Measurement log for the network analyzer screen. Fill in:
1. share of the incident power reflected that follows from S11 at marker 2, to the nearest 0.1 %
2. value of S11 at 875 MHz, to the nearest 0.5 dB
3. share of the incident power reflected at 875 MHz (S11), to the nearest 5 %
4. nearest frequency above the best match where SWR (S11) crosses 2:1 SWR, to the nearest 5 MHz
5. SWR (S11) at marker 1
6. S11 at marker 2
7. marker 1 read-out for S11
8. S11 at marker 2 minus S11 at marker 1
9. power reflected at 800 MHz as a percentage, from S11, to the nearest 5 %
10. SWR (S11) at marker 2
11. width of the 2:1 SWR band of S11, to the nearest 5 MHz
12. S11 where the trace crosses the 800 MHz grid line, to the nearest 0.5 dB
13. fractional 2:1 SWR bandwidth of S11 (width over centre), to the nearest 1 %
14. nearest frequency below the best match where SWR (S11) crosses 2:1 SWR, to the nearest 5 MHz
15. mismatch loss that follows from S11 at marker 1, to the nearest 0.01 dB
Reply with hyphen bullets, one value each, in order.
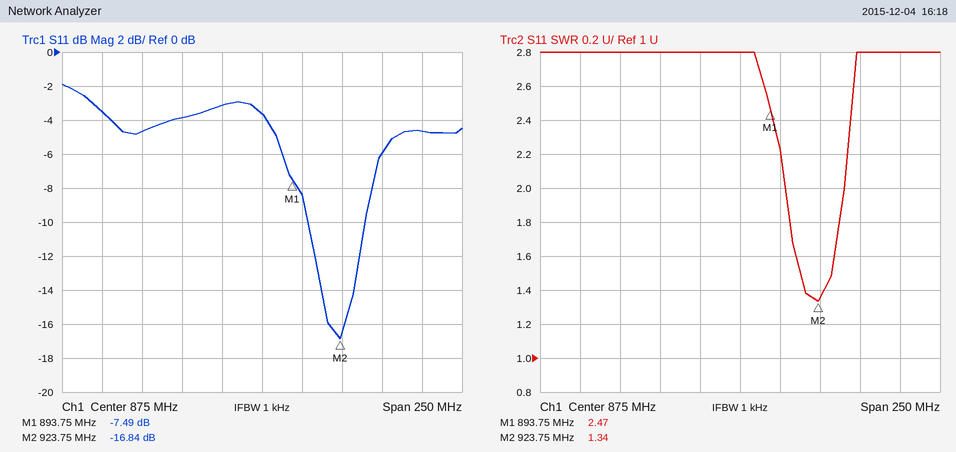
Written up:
- 2.1 %
- -3.5 dB
- 45 %
- 940 MHz
- 2.47
- -16.84 dB
- -7.49 dB
- -9.35 dB
- 35 %
- 1.34
- 35 MHz
- -4.5 dB
- 4 %
- 905 MHz
- 0.85 dB
